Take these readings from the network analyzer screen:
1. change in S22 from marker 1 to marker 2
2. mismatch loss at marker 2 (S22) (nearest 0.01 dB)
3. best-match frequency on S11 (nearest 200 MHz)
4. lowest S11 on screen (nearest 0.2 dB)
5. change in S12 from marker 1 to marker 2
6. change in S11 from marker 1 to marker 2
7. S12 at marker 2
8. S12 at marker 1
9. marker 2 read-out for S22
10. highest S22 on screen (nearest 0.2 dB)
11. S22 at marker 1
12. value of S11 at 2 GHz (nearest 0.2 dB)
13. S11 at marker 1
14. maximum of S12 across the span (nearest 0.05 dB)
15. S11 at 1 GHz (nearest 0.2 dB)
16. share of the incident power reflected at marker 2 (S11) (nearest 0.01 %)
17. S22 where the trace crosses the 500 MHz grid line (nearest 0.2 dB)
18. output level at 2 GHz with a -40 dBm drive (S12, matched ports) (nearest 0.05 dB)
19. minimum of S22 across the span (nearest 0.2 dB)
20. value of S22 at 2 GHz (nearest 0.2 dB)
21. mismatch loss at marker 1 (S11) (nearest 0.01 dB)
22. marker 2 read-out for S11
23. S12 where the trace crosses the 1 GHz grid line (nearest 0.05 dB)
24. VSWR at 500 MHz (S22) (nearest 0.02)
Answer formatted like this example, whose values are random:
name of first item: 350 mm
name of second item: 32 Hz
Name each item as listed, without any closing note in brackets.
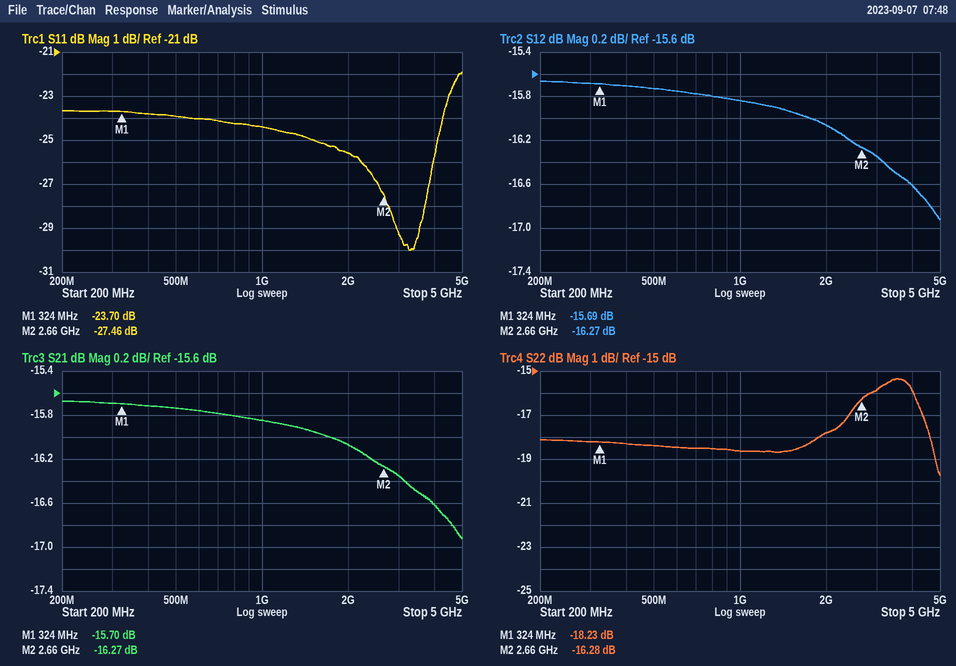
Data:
change in S22 from marker 1 to marker 2: 1.95 dB
mismatch loss at marker 2 (S22): 0.10 dB
best-match frequency on S11: 3.2 GHz
lowest S11 on screen: -30.0 dB
change in S12 from marker 1 to marker 2: -0.58 dB
change in S11 from marker 1 to marker 2: -3.76 dB
S12 at marker 2: -16.27 dB
S12 at marker 1: -15.69 dB
marker 2 read-out for S22: -16.28 dB
highest S22 on screen: -15.4 dB
S22 at marker 1: -18.23 dB
value of S11 at 2 GHz: -25.6 dB
S11 at marker 1: -23.70 dB
maximum of S12 across the span: -15.65 dB
S11 at 1 GHz: -24.4 dB
share of the incident power reflected at marker 2 (S11): 0.18 %
S22 where the trace crosses the 500 MHz grid line: -18.4 dB
output level at 2 GHz with a -40 dBm drive (S12, matched ports): -56.05 dBm
minimum of S22 across the span: -19.8 dB
value of S22 at 2 GHz: -17.8 dB
mismatch loss at marker 1 (S11): 0.02 dB
marker 2 read-out for S11: -27.46 dB
S12 where the trace crosses the 1 GHz grid line: -15.85 dB
VSWR at 500 MHz (S22): 1.28
